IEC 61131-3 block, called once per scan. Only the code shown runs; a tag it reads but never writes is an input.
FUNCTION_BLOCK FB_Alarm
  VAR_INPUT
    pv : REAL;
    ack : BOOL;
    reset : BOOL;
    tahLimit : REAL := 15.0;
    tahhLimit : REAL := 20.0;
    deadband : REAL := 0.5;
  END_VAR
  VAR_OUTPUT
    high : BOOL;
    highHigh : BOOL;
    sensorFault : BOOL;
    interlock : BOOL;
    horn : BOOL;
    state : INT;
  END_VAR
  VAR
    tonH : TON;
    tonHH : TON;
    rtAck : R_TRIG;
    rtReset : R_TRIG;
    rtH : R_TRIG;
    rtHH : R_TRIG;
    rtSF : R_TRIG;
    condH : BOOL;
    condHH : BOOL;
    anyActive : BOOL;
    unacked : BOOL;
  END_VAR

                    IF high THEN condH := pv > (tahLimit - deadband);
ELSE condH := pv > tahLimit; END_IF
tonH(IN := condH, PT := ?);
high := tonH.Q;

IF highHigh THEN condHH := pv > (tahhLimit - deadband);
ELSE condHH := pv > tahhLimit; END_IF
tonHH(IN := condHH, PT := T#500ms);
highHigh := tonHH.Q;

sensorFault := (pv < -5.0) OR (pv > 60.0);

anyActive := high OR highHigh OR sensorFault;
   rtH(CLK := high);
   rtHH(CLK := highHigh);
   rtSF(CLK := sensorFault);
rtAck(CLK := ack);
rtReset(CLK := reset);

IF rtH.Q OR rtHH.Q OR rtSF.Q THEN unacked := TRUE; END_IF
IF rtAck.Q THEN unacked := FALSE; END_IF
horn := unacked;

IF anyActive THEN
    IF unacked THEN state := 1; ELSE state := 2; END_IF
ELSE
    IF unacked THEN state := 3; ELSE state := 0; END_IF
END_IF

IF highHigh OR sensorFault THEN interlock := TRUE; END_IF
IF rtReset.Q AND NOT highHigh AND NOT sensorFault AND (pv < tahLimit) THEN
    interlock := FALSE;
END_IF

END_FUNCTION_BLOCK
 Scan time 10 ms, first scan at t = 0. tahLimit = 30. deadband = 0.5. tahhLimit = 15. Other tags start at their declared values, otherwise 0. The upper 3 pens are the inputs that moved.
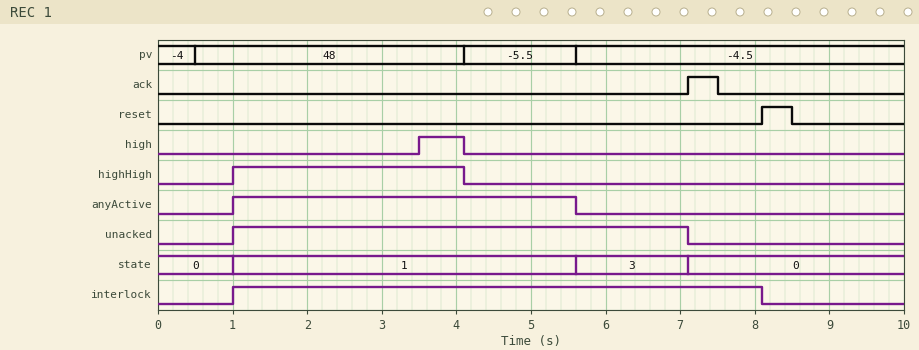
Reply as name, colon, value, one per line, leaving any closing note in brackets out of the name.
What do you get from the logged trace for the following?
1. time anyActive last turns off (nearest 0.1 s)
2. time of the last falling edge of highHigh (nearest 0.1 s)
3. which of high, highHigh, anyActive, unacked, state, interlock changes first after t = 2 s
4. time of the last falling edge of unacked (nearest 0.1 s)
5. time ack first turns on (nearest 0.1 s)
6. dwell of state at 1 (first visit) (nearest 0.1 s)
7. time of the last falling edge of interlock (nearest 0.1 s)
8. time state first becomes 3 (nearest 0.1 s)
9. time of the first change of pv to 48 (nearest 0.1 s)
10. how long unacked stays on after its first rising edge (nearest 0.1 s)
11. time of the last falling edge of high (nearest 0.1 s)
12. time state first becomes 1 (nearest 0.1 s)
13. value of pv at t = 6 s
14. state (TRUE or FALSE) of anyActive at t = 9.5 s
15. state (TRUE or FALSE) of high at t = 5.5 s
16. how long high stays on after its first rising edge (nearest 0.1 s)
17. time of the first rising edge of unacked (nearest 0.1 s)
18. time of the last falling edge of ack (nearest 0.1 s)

time anyActive last turns off: 5.6 s
time of the last falling edge of highHigh: 4.1 s
which of high, highHigh, anyActive, unacked, state, interlock changes first after t = 2 s: high
time of the last falling edge of unacked: 7.1 s
time ack first turns on: 7.1 s
dwell of state at 1 (first visit): 4.6 s
time of the last falling edge of interlock: 8.1 s
time state first becomes 3: 5.6 s
time of the first change of pv to 48: 0.5 s
how long unacked stays on after its first rising edge: 6.1 s
time of the last falling edge of high: 4.1 s
time state first becomes 1: 1.0 s
value of pv at t = 6 s: -4.5
state (TRUE or FALSE) of anyActive at t = 9.5 s: FALSE
state (TRUE or FALSE) of high at t = 5.5 s: FALSE
how long high stays on after its first rising edge: 0.6 s
time of the first rising edge of unacked: 1.0 s
time of the last falling edge of ack: 7.5 s
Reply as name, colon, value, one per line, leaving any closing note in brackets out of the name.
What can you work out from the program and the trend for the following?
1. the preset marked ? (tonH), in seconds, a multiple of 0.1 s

the preset marked ? (tonH), in seconds, a multiple of 0.1 s: 3.0 s
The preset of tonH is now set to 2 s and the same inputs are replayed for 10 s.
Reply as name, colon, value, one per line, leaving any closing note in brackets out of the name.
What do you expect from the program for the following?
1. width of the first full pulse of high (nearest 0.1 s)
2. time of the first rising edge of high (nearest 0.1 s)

width of the first full pulse of high: 1.6 s
time of the first rising edge of high: 2.5 s
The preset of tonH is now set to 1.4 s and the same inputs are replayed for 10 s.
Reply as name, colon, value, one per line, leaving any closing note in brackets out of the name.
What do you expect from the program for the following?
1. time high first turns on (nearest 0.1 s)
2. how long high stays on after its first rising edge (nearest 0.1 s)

time high first turns on: 1.9 s
how long high stays on after its first rising edge: 2.2 s
